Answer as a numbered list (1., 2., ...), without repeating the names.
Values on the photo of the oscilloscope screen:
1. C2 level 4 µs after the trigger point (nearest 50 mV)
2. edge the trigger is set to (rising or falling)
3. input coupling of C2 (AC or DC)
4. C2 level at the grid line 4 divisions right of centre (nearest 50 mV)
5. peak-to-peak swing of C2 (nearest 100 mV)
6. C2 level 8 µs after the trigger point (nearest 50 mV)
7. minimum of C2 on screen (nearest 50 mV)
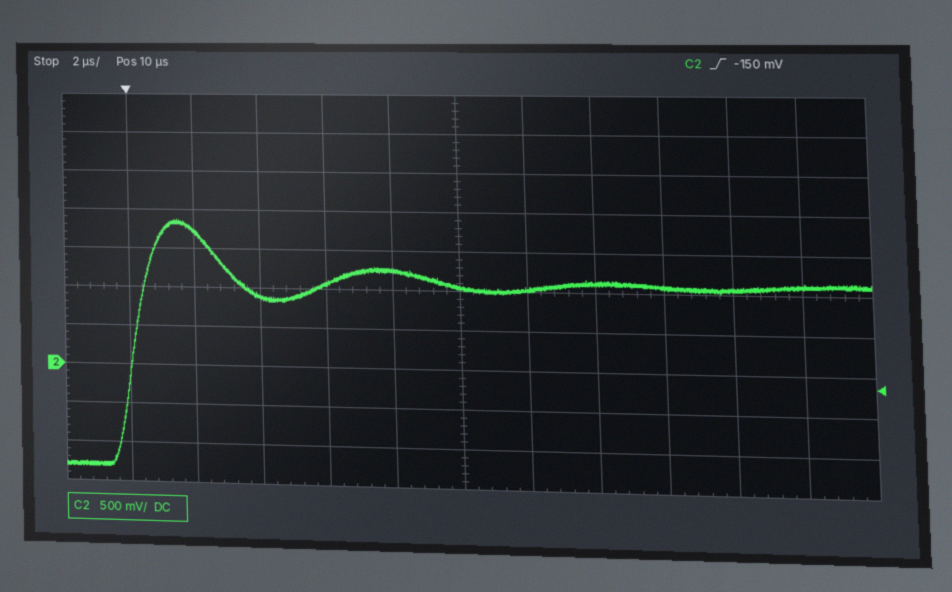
1. 900 mV
2. rising
3. DC
4. 1.05 V
5. 3.20 V
6. 1.25 V
7. -1.30 V
